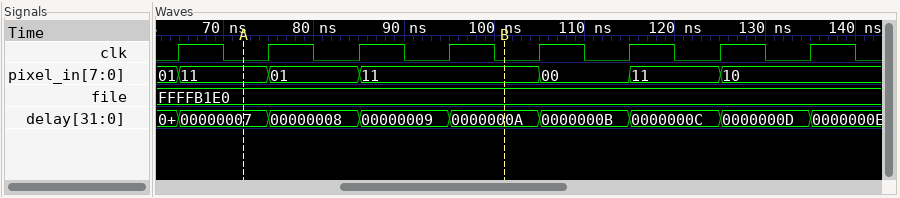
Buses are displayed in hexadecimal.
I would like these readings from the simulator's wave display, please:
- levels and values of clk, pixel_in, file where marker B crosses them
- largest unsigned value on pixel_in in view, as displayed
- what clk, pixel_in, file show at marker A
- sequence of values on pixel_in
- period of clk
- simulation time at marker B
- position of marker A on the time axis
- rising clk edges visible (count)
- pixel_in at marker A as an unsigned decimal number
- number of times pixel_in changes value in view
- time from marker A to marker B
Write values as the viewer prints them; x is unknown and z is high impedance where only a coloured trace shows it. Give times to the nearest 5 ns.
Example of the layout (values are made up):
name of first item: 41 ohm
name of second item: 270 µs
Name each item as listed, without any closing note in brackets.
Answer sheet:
levels and values of clk, pixel_in, file where marker B crosses them: clk=0, pixel_in=11, file=FFFFB1E0
largest unsigned value on pixel_in in view, as displayed: 11
what clk, pixel_in, file show at marker A: clk=0, pixel_in=11, file=FFFFB1E0
sequence of values on pixel_in: 01, 11, 01, 11, 00, 11, 10
period of clk: 10 ns
simulation time at marker B: 100 ns
position of marker A on the time axis: 70 ns
rising clk edges visible: 8
pixel_in at marker A as an unsigned decimal number: 17
number of times pixel_in changes value in view: 6
time from marker A to marker B: 30 ns
